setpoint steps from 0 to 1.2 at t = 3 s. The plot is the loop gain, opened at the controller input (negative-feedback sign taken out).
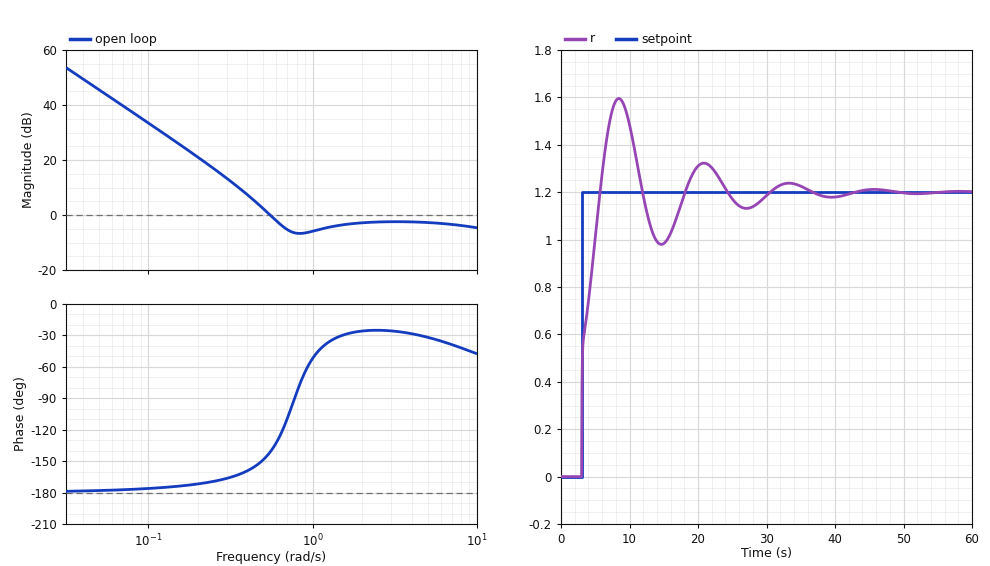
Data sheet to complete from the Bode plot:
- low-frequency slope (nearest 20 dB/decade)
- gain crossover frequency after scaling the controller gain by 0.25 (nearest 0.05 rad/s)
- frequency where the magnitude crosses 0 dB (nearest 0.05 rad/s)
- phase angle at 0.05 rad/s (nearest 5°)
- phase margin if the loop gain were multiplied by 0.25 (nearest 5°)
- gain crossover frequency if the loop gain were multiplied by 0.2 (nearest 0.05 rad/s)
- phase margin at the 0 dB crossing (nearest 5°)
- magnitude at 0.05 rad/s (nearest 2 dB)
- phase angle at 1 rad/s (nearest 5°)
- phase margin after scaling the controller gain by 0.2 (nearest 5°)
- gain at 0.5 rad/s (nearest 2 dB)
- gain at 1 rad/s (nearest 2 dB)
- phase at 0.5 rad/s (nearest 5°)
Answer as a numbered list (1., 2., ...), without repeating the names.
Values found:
1. -40 dB/decade
2. 0.30 rad/s
3. 0.55 rad/s
4. -180°
5. 15°
6. 0.30 rad/s
7. 40°
8. 46 dB
9. -50°
10. 15°
11. 2 dB
12. -6 dB
13. -150°
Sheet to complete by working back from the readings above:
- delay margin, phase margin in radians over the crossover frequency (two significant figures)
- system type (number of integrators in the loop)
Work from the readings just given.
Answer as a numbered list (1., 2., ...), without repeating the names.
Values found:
1. 1.3 s
2. 2
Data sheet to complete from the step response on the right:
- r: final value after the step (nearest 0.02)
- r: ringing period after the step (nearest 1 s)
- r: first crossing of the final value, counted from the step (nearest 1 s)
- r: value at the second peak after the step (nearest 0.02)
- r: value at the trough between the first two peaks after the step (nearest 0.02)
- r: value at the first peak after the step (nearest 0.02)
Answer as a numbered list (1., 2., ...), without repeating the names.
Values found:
1. 1.20
2. 12 s
3. 3 s
4. 1.32
5. 0.98
6. 1.60
